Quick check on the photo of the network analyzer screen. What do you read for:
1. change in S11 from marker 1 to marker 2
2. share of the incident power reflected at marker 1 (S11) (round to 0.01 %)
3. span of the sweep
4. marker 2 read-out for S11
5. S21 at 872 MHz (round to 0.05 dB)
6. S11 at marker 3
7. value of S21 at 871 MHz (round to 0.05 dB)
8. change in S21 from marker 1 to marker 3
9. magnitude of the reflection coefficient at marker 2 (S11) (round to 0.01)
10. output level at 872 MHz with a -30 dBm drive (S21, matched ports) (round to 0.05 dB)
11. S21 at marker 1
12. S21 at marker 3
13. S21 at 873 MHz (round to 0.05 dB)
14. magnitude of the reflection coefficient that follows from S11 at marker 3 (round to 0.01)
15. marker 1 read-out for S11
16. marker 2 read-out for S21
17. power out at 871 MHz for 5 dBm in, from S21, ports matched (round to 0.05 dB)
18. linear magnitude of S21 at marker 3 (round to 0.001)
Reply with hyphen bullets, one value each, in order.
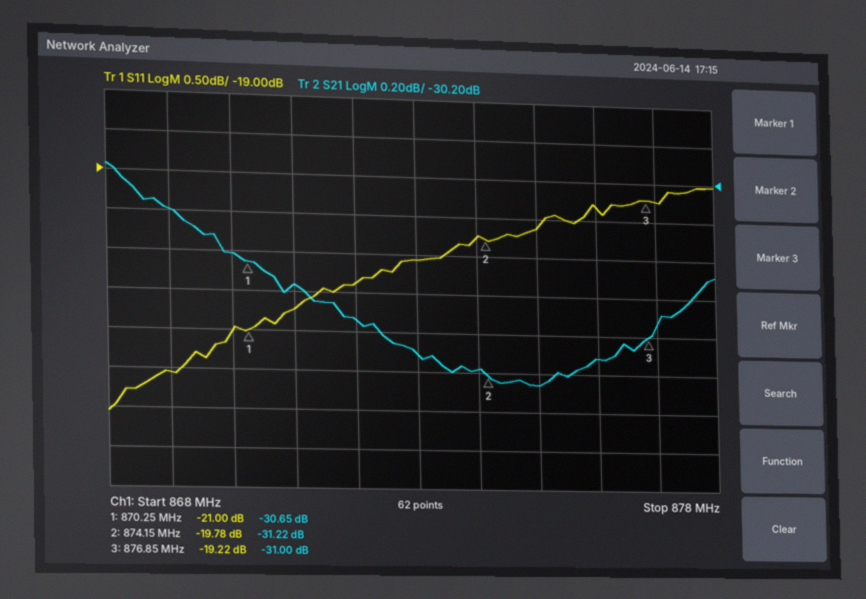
- 1.22 dB
- 0.79 %
- 10 MHz
- -19.78 dB
- -30.95 dB
- -19.22 dB
- -30.75 dB
- -0.35 dB
- 0.10
- -60.95 dBm
- -30.65 dB
- -31.00 dB
- -31.10 dB
- 0.11
- -21.00 dB
- -31.22 dB
- -25.75 dBm
- 0.028
